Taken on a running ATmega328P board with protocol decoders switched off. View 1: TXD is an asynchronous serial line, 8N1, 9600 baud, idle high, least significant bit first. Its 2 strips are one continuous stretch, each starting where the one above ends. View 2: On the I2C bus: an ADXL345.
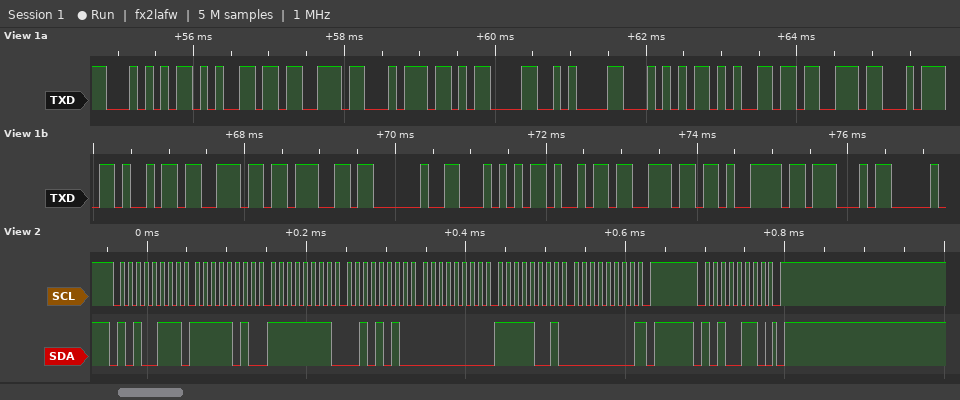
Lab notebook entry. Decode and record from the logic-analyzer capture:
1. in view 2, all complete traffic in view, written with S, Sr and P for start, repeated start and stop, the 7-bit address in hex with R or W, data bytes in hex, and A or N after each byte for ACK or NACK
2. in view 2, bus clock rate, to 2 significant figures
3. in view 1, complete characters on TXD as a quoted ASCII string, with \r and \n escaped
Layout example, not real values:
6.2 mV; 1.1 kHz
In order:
S 53R A FA A FF A 2A A 00 A F9 A 00 N P S 53W A P; 100 kHz; "Test\r\nTesting TinyG"
